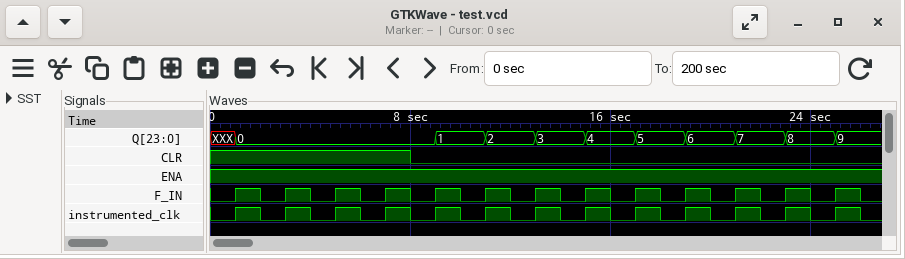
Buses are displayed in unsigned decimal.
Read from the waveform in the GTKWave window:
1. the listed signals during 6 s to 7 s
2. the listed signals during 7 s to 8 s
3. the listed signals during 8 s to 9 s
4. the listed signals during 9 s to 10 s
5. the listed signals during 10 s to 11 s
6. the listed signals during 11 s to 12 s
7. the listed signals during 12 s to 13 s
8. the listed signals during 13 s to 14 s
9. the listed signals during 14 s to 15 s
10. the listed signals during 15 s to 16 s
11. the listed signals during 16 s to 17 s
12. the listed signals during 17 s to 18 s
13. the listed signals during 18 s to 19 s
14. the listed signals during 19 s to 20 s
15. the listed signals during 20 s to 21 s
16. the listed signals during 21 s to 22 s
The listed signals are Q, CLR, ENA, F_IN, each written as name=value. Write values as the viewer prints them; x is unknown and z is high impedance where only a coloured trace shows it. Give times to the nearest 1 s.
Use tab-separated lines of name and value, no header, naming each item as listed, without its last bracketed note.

the listed signals during 6 s to 7 s	Q=0, CLR=1, ENA=1, F_IN=0
the listed signals during 7 s to 8 s	Q=0, CLR=1, ENA=1, F_IN=1
the listed signals during 8 s to 9 s	Q=0, CLR=0, ENA=1, F_IN=0
the listed signals during 9 s to 10 s	Q=1, CLR=0, ENA=1, F_IN=1
the listed signals during 10 s to 11 s	Q=1, CLR=0, ENA=1, F_IN=0
the listed signals during 11 s to 12 s	Q=2, CLR=0, ENA=1, F_IN=1
the listed signals during 12 s to 13 s	Q=2, CLR=0, ENA=1, F_IN=0
the listed signals during 13 s to 14 s	Q=3, CLR=0, ENA=1, F_IN=1
the listed signals during 14 s to 15 s	Q=3, CLR=0, ENA=1, F_IN=0
the listed signals during 15 s to 16 s	Q=4, CLR=0, ENA=1, F_IN=1
the listed signals during 16 s to 17 s	Q=4, CLR=0, ENA=1, F_IN=0
the listed signals during 17 s to 18 s	Q=5, CLR=0, ENA=1, F_IN=1
the listed signals during 18 s to 19 s	Q=5, CLR=0, ENA=1, F_IN=0
the listed signals during 19 s to 20 s	Q=6, CLR=0, ENA=1, F_IN=1
the listed signals during 20 s to 21 s	Q=6, CLR=0, ENA=1, F_IN=0
the listed signals during 21 s to 22 s	Q=7, CLR=0, ENA=1, F_IN=1
